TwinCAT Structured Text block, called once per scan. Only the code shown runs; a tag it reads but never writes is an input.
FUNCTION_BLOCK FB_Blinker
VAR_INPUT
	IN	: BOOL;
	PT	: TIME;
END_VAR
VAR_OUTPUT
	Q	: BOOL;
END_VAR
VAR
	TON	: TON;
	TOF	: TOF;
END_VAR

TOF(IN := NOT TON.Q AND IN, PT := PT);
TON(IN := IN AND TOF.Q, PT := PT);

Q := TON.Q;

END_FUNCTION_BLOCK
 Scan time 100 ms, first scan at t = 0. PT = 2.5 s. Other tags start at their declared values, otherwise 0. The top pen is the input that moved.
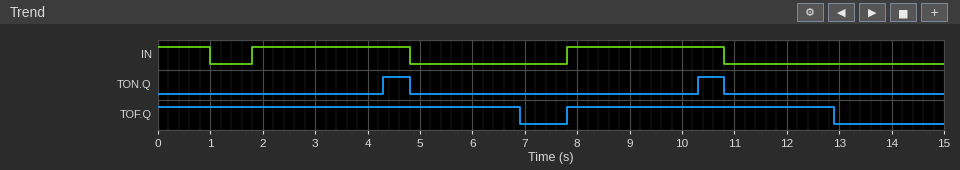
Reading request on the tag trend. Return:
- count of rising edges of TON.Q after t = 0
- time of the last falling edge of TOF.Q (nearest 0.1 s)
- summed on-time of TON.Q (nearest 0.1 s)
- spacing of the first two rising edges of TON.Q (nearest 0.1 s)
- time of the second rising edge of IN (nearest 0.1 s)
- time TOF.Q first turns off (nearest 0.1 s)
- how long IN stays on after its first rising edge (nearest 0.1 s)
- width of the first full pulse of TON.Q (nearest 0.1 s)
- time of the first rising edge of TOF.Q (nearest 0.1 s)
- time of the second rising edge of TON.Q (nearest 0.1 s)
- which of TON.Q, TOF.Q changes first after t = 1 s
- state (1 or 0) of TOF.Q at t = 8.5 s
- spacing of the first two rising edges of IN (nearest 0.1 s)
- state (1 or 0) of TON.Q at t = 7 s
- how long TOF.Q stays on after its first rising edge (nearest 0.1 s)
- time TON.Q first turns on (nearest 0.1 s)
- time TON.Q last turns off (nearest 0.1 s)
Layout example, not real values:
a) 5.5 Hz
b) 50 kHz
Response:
a) 2
b) 12.9 s
c) 1.0 s
d) 6.0 s
e) 7.8 s
f) 6.9 s
g) 3.0 s
h) 0.5 s
i) 7.8 s
j) 10.3 s
k) TON.Q
l) 1
m) 6.0 s
n) 0
o) 5.1 s
p) 4.3 s
q) 10.8 s
